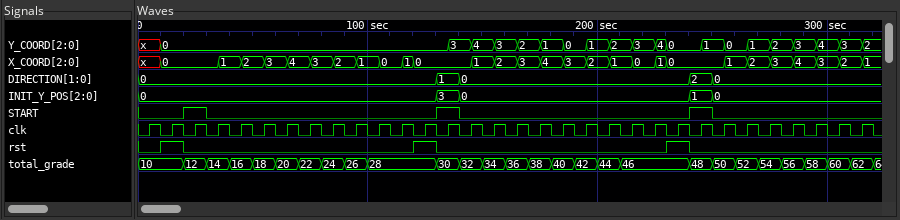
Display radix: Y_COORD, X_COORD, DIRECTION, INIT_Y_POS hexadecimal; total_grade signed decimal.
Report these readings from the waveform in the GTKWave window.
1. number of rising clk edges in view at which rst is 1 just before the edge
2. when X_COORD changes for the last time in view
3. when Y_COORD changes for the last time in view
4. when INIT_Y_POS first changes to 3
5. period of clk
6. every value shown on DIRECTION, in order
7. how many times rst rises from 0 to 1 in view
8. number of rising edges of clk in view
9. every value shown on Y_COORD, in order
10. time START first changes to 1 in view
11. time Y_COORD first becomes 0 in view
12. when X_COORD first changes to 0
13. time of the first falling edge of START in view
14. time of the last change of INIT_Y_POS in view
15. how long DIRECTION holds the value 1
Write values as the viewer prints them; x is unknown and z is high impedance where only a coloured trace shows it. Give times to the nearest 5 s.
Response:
3
315 s
315 s
130 s
10 s
0, 1, 0, 2, 0
3
32
x, 0, 3, 4, 3, 2, 1, 0, 1, 2, 3, 4, 0, 1, 0, 1, 2, 3, 4, 3, 2
20 s
10 s
10 s
30 s
250 s
10 s
